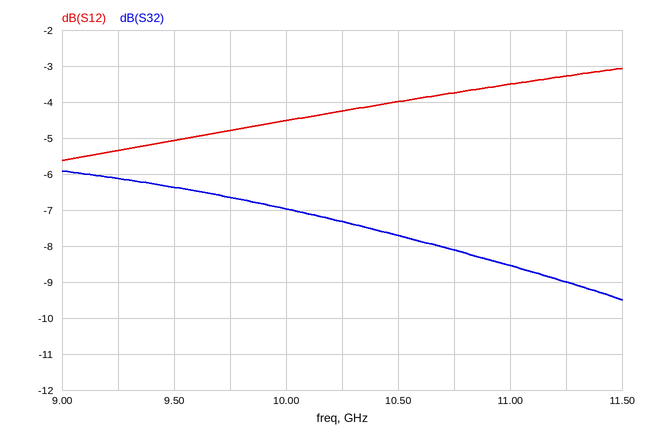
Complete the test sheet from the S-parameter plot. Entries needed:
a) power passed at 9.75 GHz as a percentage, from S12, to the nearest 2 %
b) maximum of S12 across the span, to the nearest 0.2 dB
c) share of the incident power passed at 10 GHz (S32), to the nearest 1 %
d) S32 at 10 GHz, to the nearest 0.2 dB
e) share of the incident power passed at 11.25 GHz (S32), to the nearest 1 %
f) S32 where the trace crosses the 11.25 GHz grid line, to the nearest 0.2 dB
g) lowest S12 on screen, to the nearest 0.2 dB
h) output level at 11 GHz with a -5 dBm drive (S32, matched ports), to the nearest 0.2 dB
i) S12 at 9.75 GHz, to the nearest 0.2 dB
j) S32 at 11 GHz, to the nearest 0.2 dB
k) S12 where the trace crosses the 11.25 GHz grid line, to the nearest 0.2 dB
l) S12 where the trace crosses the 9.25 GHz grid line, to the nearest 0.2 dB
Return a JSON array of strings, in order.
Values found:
["34 %", "-3.0 dB", "20 %", "-7.0 dB", "13 %", "-9.0 dB", "-5.6 dB", "-13.6 dBm", "-4.8 dB", "-8.6 dB", "-3.2 dB", "-5.4 dB"]
